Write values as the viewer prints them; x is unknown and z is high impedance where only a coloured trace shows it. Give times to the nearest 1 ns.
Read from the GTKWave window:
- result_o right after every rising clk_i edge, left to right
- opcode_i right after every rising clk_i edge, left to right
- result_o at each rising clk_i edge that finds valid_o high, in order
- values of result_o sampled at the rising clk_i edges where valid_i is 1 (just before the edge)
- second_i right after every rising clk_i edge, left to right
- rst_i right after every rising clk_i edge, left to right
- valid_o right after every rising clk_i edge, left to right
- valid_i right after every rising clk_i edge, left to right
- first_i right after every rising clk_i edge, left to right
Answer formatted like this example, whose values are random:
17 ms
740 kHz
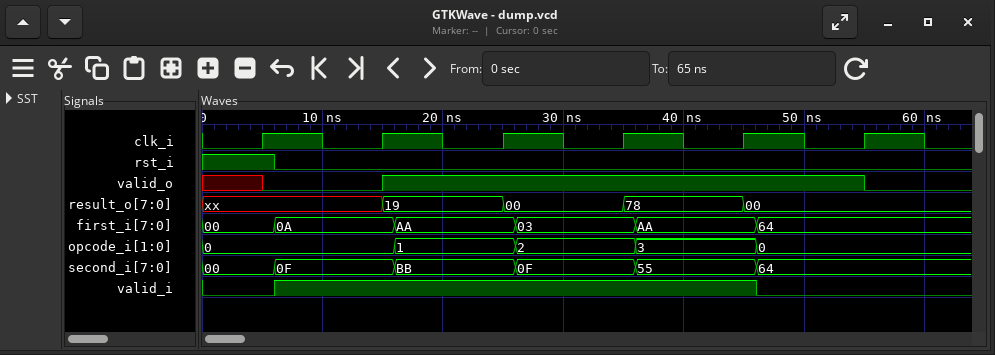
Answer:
xx, 19, 00, 78, 00, 00
0, 0, 1, 2, 3, 0
19, 00, 78, 00
xx, 19, 00, 78
00, 0F, BB, 0F, 55, 64
1 0 0 0 0 0
0 1 1 1 1 0
0 1 1 1 1 0
00, 0A, AA, 03, AA, 64
